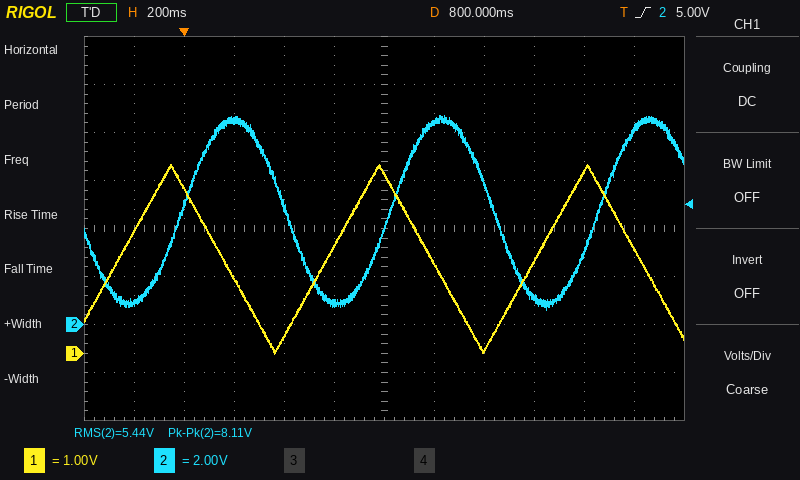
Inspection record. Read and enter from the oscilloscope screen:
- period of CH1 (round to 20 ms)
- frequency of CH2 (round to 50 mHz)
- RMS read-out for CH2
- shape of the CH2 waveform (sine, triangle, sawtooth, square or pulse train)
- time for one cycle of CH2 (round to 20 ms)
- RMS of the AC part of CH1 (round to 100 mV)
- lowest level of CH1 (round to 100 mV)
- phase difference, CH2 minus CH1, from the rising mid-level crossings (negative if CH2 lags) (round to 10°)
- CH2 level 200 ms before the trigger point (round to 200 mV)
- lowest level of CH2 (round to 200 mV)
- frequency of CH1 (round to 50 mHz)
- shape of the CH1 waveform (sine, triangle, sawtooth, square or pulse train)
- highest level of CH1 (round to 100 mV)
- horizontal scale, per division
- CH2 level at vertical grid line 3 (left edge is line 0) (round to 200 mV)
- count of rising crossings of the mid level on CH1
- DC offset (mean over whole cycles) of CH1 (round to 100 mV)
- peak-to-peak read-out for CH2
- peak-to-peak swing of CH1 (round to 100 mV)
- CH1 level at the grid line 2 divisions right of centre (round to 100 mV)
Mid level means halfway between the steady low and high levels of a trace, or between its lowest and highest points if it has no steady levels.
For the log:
840 ms
1.20 Hz
5.44 V
sine
840 ms
1.1 V
0.0 V
-110°
1.0 V
600 mV
1.20 Hz
triangle
3.9 V
200 ms
8.6 V
3
2.0 V
8.11 V
3.9 V
100 mV
